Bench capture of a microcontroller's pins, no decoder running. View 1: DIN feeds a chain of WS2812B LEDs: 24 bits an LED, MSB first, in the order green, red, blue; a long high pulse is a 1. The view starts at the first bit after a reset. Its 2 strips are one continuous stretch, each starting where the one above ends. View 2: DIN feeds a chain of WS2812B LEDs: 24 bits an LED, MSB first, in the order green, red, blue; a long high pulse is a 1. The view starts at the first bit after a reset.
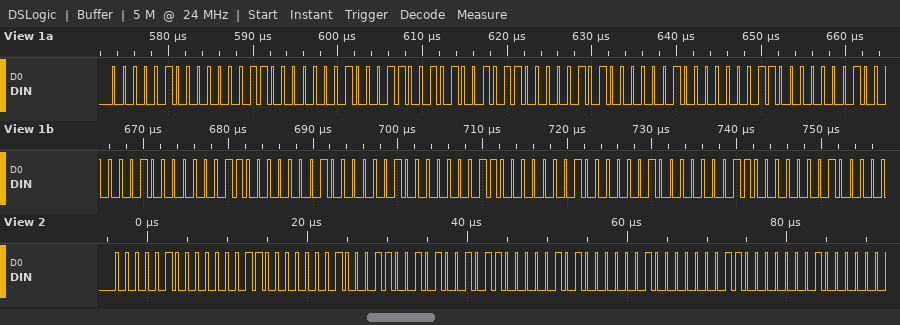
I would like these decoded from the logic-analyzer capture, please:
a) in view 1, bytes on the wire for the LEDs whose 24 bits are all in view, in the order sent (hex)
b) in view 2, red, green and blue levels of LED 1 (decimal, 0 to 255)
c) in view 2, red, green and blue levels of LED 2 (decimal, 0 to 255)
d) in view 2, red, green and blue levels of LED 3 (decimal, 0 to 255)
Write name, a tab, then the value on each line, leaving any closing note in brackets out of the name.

in view 1, bytes on the wire for the LEDs whose 24 bits are all in view, in the order sent	04 06 02 32 96 0A 04 06 02 04 06 02 04 06 02 04 06 02
in view 2, red, green and blue levels of LED 1	6, 4, 2
in view 2, red, green and blue levels of LED 2	150, 50, 10
in view 2, red, green and blue levels of LED 3	6, 4, 2
